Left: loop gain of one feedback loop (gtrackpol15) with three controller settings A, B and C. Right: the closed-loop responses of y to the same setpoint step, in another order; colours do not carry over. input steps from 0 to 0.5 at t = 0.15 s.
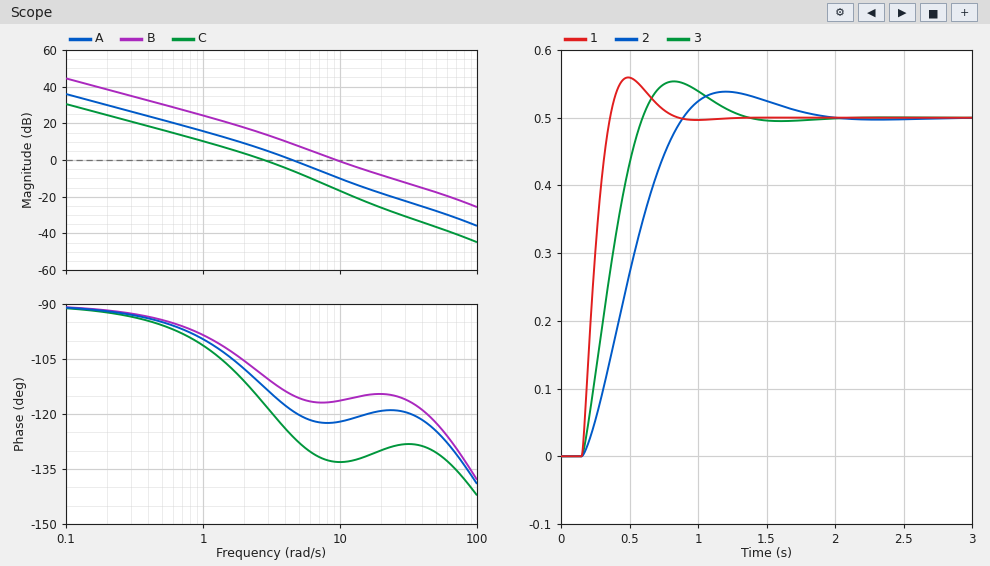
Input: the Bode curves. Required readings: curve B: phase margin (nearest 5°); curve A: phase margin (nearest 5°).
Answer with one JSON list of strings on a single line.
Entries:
["65°", "60°"]
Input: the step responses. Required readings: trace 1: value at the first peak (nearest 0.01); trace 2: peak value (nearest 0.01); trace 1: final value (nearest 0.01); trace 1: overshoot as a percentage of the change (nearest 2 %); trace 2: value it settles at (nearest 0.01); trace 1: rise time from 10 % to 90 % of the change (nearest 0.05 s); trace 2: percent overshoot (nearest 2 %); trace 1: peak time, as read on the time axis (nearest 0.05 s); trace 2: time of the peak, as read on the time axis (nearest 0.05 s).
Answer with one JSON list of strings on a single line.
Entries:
["0.56", "0.54", "0.50", "12 %", "0.50", "0.15 s", "8 %", "0.50 s", "1.20 s"]
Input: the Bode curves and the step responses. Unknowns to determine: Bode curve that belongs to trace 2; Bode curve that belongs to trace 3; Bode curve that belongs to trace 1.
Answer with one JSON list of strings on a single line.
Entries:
["C", "A", "B"]
